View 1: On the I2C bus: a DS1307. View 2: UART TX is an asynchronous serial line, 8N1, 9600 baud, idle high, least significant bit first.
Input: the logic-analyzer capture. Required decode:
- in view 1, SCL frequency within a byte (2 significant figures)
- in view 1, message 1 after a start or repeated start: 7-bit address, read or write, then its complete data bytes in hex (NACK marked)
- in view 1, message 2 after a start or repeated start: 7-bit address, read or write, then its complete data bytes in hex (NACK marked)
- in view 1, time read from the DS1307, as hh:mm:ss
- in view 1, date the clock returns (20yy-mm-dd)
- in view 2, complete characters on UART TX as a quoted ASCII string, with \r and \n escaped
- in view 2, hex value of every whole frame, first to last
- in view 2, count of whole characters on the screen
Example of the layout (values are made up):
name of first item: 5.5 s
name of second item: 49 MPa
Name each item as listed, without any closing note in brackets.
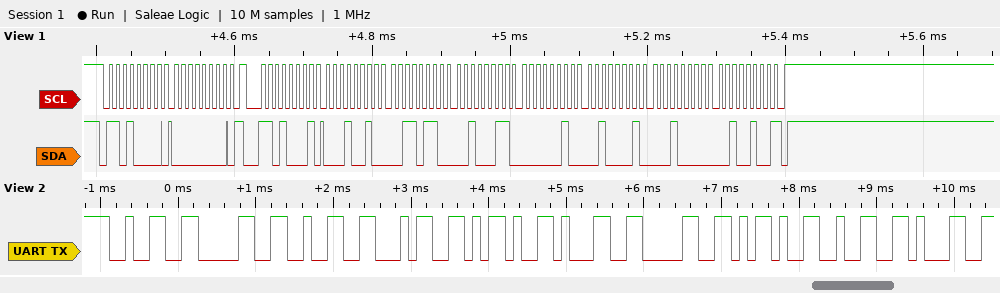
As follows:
in view 1, SCL frequency within a byte: 100 kHz
in view 1, message 1 after a start or repeated start: 7-bit address, read or write, then its complete data bytes in hex: 0x68 write: 00
in view 1, message 2 after a start or repeated start: 7-bit address, read or write, then its complete data bytes in hex: 0x68 read: 12 36 23 02 21 10 24 NACK
in view 1, time read from the DS1307, as hh:mm:ss: 23:36:12
in view 1, date the clock returns: 2024-10-21
in view 2, complete characters on UART TX as a quoted ASCII string, with \r and \n escaped: "2024-10-21"
in view 2, hex value of every whole frame, first to last: 32 30 32 34 2D 31 30 2D 32 31
in view 2, count of whole characters on the screen: 10
